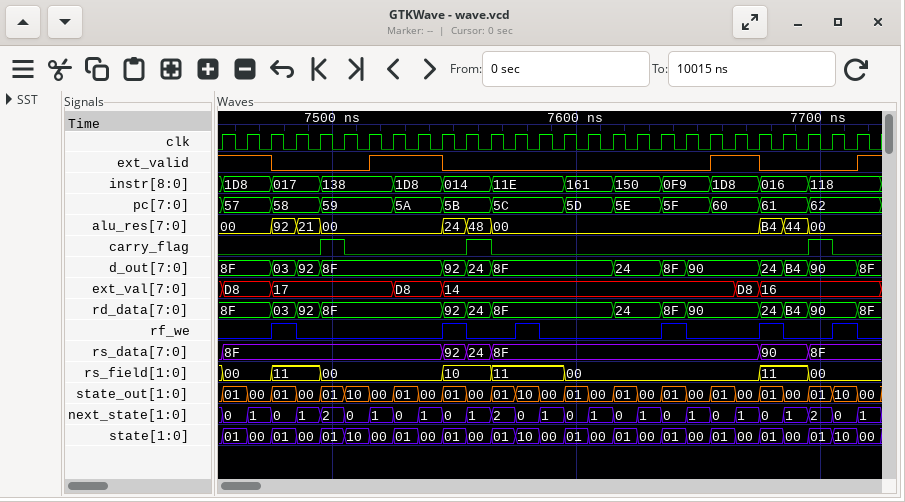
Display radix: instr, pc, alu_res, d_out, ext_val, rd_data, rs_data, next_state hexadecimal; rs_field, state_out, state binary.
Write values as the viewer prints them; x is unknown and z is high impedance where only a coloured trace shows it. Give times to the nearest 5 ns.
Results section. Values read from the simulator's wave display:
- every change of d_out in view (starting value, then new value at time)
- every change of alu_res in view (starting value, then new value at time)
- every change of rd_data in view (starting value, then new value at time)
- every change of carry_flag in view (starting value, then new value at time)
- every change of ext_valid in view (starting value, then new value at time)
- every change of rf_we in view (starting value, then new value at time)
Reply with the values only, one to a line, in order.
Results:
8F, 03 at 7475 ns, 92 at 7485 ns, 8F at 7495 ns, 92 at 7545 ns, 24 at 7555 ns, 8F at 7565 ns, 24 at 7615 ns, 8F at 7635 ns, 90 at 7645 ns, 24 at 7675 ns, B4 at 7685 ns, 90 at 7695 ns, 8F at 7715 ns
00, 92 at 7475 ns, 21 at 7485 ns, 00 at 7495 ns, 24 at 7545 ns, 48 at 7555 ns, 00 at 7565 ns, B4 at 7675 ns, 44 at 7685 ns, 00 at 7695 ns
8F, 03 at 7475 ns, 92 at 7485 ns, 8F at 7495 ns, 92 at 7545 ns, 24 at 7555 ns, 8F at 7565 ns, 24 at 7615 ns, 8F at 7635 ns, 90 at 7645 ns, 24 at 7675 ns, B4 at 7685 ns, 90 at 7695 ns, 8F at 7715 ns
0, 1 at 7495 ns, 0 at 7505 ns, 1 at 7555 ns, 0 at 7565 ns, 1 at 7695 ns, 0 at 7705 ns
1, 0 at 7475 ns, 1 at 7515 ns, 0 at 7545 ns, 1 at 7655 ns, 0 at 7675 ns, 1 at 7715 ns
0, 1 at 7475 ns, 0 at 7485 ns, 1 at 7545 ns, 0 at 7555 ns, 1 at 7575 ns, 0 at 7585 ns, 1 at 7635 ns, 0 at 7645 ns, 1 at 7675 ns, 0 at 7685 ns, 1 at 7705 ns, 0 at 7715 ns
